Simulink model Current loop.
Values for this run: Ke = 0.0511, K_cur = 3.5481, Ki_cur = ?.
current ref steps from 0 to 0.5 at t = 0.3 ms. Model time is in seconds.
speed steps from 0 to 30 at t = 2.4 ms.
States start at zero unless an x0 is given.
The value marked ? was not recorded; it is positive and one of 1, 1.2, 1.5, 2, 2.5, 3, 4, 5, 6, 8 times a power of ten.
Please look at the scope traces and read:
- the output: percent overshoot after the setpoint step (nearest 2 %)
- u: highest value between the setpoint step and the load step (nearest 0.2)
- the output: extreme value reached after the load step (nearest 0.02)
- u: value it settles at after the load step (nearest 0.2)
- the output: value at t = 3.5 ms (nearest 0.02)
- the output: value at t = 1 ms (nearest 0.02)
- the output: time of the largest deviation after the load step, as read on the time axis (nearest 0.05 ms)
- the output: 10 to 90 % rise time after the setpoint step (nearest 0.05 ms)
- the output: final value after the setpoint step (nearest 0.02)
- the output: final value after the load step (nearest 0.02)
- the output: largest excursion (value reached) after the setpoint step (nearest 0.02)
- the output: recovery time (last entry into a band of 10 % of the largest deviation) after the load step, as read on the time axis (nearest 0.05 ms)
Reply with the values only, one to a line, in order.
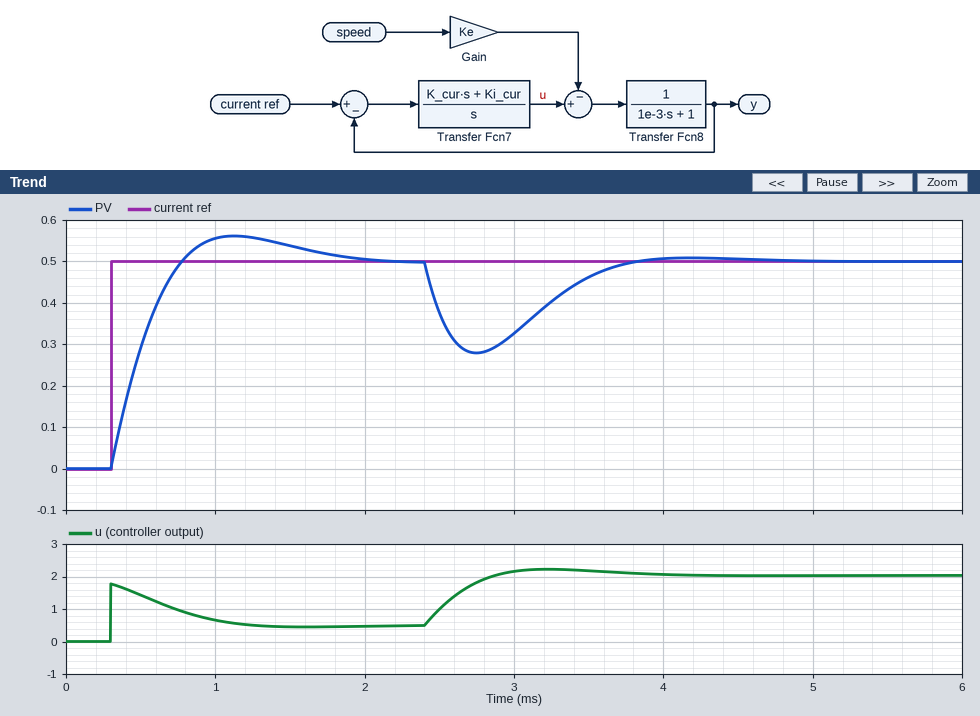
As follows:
12 %
1.8
0.28
2.0
0.46
0.56
2.75 ms
0.35 ms
0.50
0.50
0.56
3.60 ms
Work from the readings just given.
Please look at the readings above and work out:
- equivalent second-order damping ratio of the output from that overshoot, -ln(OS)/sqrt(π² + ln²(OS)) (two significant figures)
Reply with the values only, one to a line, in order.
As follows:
0.56
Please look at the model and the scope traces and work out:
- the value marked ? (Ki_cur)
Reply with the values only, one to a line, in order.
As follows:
10000
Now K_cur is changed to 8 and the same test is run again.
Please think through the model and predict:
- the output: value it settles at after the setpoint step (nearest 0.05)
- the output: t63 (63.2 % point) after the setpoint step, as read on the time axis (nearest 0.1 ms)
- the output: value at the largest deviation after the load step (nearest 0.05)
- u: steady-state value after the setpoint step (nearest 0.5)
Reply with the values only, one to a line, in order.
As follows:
0.50
0.4 ms
0.35
0.5
